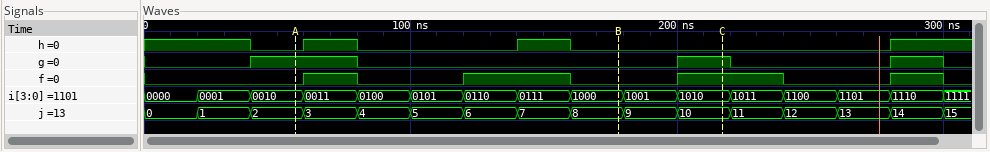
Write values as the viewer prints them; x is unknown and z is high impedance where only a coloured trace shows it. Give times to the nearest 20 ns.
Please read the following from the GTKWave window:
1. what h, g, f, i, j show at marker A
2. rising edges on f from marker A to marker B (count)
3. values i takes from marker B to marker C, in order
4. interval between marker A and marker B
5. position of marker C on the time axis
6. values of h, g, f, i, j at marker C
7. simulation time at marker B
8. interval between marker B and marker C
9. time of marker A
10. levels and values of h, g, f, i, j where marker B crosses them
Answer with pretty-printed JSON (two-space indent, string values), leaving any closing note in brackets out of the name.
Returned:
{
  "what h, g, f, i, j show at marker A": "h=0, g=1, f=0, i=0010, j=2",
  "rising edges on f from marker A to marker B": "2",
  "values i takes from marker B to marker C, in order": "1000, 1001, 1010",
  "interval between marker A and marker B": "120 ns",
  "position of marker C on the time axis": "220 ns",
  "values of h, g, f, i, j at marker C": "h=0, g=1, f=1, i=1010, j=10",
  "simulation time at marker B": "180 ns",
  "interval between marker B and marker C": "40 ns",
  "time of marker A": "60 ns",
  "levels and values of h, g, f, i, j where marker B crosses them": "h=0, g=0, f=0, i=1000, j=8"
}
